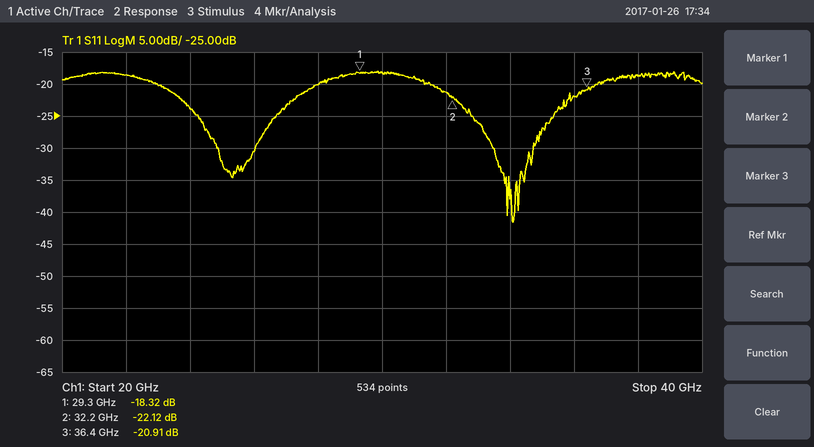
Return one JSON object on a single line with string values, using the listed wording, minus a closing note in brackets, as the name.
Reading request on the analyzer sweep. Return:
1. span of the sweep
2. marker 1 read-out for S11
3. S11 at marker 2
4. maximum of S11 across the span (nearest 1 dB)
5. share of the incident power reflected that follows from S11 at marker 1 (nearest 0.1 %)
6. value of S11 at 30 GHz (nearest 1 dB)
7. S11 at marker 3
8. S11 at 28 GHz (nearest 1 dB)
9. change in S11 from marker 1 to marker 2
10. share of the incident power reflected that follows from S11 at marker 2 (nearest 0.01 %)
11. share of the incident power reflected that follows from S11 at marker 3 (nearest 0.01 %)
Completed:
{"span of the sweep": "20 GHz", "marker 1 read-out for S11": "-18.32 dB", "S11 at marker 2": "-22.12 dB", "maximum of S11 across the span": "-18 dB", "share of the incident power reflected that follows from S11 at marker 1": "1.5 %", "value of S11 at 30 GHz": "-18 dB", "S11 at marker 3": "-20.91 dB", "S11 at 28 GHz": "-20 dB", "change in S11 from marker 1 to marker 2": "-3.80 dB", "share of the incident power reflected that follows from S11 at marker 2": "0.61 %", "share of the incident power reflected that follows from S11 at marker 3": "0.81 %"}
